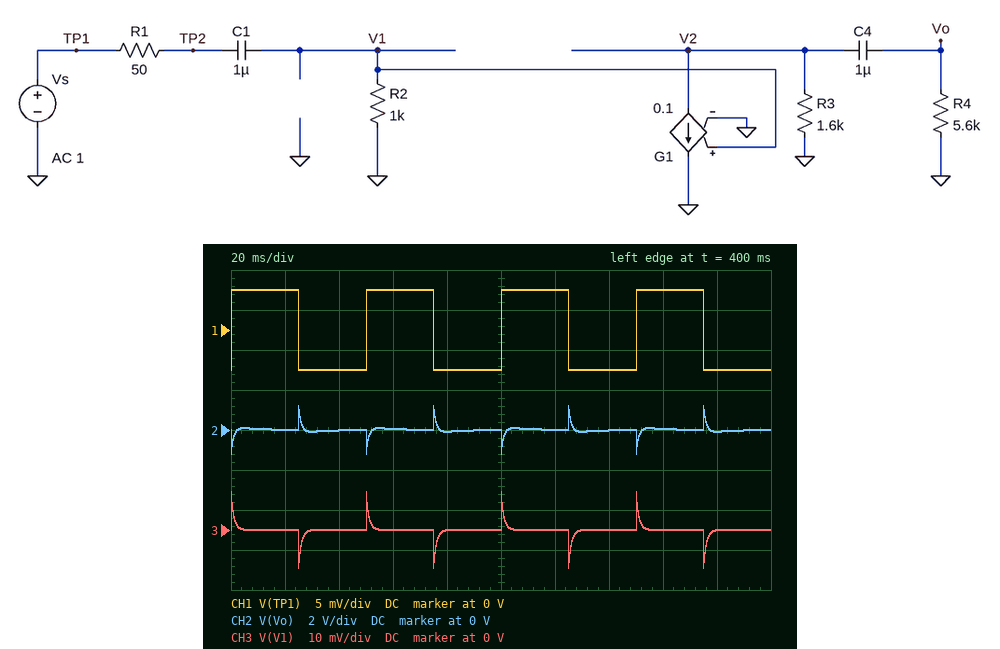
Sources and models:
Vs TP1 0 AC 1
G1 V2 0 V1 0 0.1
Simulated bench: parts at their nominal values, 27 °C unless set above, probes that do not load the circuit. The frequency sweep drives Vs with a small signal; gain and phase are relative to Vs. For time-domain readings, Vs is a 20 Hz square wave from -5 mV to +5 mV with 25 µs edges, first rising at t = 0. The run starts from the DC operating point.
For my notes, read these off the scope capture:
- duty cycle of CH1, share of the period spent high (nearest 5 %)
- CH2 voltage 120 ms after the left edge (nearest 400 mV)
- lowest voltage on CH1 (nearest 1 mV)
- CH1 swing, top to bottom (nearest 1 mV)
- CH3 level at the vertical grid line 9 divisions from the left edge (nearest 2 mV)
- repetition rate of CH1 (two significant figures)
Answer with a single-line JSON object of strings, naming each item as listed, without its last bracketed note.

{"duty cycle of CH1, share of the period spent high": "50 %", "CH2 voltage 120 ms after the left edge": "0 V", "lowest voltage on CH1": "-5 mV", "CH1 swing, top to bottom": "10 mV", "CH3 level at the vertical grid line 9 divisions from the left edge": "0 V", "repetition rate of CH1": "20 Hz"}
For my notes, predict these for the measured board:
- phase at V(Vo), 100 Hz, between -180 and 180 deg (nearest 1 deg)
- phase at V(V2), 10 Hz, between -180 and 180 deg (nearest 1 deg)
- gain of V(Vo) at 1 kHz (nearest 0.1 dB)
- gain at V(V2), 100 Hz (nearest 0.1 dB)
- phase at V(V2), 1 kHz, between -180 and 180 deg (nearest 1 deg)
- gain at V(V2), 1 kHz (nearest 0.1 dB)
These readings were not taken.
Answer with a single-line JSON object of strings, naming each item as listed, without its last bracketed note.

{"phase at V(Vo), 100 Hz, between -180 and 180 deg": "-111 deg", "phase at V(V2), 10 Hz, between -180 and 180 deg": "-99 deg", "gain of V(Vo) at 1 kHz": "41.4 dB", "gain at V(V2), 100 Hz": "36.4 dB", "phase at V(V2), 1 kHz, between -180 and 180 deg": "-172 deg", "gain at V(V2), 1 kHz": "41.4 dB"}
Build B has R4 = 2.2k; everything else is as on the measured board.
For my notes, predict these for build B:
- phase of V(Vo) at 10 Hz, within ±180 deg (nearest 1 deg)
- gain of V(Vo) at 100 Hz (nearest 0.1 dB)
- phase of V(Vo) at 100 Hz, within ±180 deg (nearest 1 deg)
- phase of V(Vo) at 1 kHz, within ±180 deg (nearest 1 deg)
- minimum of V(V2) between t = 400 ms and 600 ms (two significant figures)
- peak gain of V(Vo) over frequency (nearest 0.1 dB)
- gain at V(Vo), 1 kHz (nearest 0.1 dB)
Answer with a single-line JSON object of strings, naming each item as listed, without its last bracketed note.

{"phase of V(Vo) at 10 Hz, within ±180 deg": "-17 deg", "gain of V(Vo) at 100 Hz": "33.0 dB", "phase of V(Vo) at 100 Hz, within ±180 deg": "-101 deg", "phase of V(Vo) at 1 kHz, within ±180 deg": "-169 deg", "minimum of V(V2) between t = 400 ms and 600 ms": "-870 mV", "peak gain of V(Vo) over frequency": "38.9 dB", "gain at V(Vo), 1 kHz": "38.8 dB"}
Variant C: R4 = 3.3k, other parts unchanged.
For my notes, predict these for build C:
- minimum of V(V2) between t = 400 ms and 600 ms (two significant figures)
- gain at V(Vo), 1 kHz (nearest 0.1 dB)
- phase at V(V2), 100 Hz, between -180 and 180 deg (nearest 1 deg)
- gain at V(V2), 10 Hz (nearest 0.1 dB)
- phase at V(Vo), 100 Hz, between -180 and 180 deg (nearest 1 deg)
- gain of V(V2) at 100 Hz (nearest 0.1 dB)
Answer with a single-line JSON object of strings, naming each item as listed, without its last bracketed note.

{"minimum of V(V2) between t = 400 ms and 600 ms": "-1.0 V", "gain at V(Vo), 1 kHz": "40.1 dB", "phase at V(V2), 100 Hz, between -180 and 180 deg": "-131 deg", "gain at V(V2), 10 Hz": "19.8 dB", "phase at V(Vo), 100 Hz, between -180 and 180 deg": "-105 deg", "gain of V(V2) at 100 Hz": "35.5 dB"}
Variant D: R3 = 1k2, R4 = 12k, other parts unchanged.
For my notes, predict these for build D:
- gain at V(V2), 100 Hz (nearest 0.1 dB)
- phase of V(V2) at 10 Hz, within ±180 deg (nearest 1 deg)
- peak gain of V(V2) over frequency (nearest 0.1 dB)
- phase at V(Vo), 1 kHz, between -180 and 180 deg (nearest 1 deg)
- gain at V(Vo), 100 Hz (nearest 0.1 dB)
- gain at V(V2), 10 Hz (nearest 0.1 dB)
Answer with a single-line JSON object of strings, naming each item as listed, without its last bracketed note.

{"gain at V(V2), 100 Hz": "35.2 dB", "phase of V(V2) at 10 Hz, within ±180 deg": "-96 deg", "peak gain of V(V2) over frequency": "40.3 dB", "phase at V(Vo), 1 kHz, between -180 and 180 deg": "-171 deg", "gain at V(Vo), 100 Hz": "35.1 dB", "gain at V(V2), 10 Hz": "17.2 dB"}
